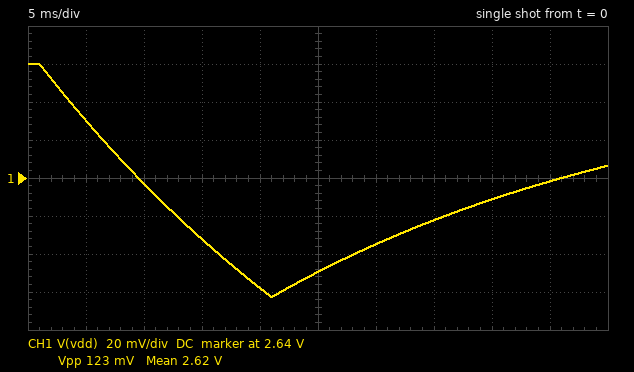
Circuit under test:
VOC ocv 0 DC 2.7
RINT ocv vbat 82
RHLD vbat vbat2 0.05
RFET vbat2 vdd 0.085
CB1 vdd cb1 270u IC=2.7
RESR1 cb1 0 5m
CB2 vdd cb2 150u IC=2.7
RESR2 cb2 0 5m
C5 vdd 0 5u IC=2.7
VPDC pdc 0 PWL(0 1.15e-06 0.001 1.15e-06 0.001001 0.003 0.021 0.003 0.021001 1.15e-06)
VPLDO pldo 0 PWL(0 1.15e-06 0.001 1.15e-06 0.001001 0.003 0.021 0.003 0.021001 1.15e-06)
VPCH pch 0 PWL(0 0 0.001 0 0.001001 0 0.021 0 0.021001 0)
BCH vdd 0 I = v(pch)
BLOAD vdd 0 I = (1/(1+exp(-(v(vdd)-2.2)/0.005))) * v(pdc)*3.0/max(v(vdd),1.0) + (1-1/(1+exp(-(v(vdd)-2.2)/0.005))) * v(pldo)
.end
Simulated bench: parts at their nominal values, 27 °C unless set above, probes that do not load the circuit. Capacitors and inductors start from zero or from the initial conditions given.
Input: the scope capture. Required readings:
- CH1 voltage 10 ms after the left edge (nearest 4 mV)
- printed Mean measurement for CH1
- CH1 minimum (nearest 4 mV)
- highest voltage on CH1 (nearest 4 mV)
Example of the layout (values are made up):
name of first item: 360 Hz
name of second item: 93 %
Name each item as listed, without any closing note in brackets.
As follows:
CH1 voltage 10 ms after the left edge: 2.636 V
printed Mean measurement for CH1: 2.62 V
CH1 minimum: 2.576 V
highest voltage on CH1: 2.700 V
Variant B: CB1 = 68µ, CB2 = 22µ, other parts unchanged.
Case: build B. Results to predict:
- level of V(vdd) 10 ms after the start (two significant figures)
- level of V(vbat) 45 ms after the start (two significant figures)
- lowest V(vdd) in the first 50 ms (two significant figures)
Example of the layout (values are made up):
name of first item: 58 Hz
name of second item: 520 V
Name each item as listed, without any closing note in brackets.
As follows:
level of V(vdd) 10 ms after the start: 2.5 V
level of V(vbat) 45 ms after the start: 2.7 V
lowest V(vdd) in the first 50 ms: 2.4 V
